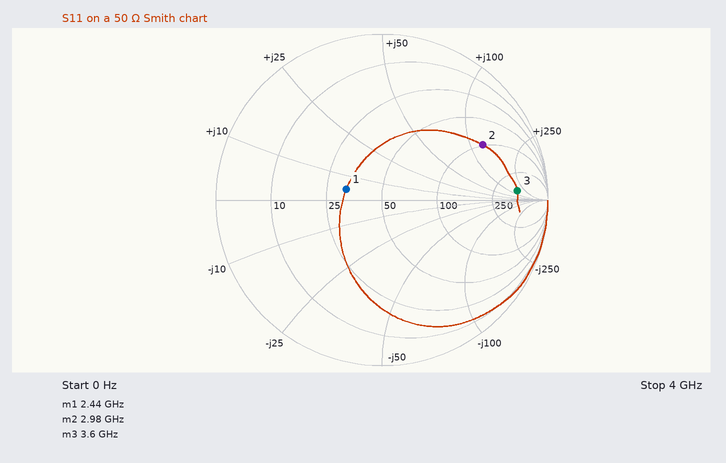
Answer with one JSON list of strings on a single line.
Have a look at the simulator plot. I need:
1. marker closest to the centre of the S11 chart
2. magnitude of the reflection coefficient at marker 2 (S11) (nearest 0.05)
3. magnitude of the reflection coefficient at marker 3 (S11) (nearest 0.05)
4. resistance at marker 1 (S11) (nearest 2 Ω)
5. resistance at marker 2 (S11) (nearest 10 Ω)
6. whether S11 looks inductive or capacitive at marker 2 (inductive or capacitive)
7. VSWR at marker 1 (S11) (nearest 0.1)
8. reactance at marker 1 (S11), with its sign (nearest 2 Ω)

["marker 1", "0.70", "0.80", "32 Ω", "100 Ω", "inductive", "1.6", "+4 Ω"]
